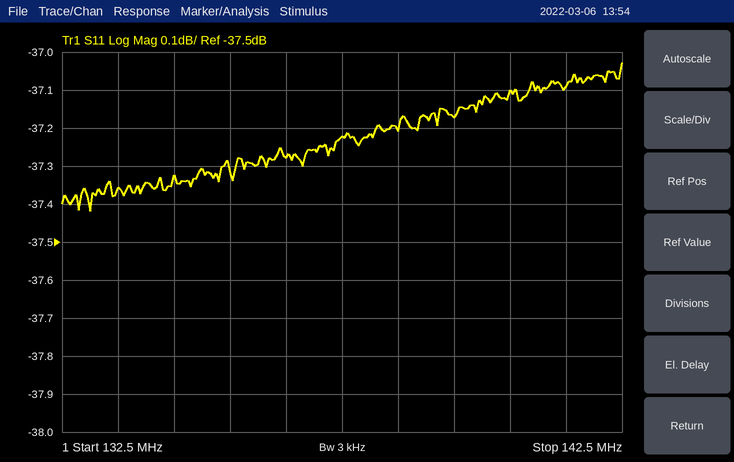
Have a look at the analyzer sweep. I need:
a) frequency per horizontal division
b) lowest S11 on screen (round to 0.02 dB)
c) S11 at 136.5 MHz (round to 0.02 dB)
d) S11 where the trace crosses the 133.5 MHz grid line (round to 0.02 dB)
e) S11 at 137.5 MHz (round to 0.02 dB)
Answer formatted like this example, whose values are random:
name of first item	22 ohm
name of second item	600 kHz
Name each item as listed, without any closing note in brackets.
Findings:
frequency per horizontal division	1 MHz
lowest S11 on screen	-37.42 dB
S11 at 136.5 MHz	-37.28 dB
S11 where the trace crosses the 133.5 MHz grid line	-37.36 dB
S11 at 137.5 MHz	-37.22 dB
